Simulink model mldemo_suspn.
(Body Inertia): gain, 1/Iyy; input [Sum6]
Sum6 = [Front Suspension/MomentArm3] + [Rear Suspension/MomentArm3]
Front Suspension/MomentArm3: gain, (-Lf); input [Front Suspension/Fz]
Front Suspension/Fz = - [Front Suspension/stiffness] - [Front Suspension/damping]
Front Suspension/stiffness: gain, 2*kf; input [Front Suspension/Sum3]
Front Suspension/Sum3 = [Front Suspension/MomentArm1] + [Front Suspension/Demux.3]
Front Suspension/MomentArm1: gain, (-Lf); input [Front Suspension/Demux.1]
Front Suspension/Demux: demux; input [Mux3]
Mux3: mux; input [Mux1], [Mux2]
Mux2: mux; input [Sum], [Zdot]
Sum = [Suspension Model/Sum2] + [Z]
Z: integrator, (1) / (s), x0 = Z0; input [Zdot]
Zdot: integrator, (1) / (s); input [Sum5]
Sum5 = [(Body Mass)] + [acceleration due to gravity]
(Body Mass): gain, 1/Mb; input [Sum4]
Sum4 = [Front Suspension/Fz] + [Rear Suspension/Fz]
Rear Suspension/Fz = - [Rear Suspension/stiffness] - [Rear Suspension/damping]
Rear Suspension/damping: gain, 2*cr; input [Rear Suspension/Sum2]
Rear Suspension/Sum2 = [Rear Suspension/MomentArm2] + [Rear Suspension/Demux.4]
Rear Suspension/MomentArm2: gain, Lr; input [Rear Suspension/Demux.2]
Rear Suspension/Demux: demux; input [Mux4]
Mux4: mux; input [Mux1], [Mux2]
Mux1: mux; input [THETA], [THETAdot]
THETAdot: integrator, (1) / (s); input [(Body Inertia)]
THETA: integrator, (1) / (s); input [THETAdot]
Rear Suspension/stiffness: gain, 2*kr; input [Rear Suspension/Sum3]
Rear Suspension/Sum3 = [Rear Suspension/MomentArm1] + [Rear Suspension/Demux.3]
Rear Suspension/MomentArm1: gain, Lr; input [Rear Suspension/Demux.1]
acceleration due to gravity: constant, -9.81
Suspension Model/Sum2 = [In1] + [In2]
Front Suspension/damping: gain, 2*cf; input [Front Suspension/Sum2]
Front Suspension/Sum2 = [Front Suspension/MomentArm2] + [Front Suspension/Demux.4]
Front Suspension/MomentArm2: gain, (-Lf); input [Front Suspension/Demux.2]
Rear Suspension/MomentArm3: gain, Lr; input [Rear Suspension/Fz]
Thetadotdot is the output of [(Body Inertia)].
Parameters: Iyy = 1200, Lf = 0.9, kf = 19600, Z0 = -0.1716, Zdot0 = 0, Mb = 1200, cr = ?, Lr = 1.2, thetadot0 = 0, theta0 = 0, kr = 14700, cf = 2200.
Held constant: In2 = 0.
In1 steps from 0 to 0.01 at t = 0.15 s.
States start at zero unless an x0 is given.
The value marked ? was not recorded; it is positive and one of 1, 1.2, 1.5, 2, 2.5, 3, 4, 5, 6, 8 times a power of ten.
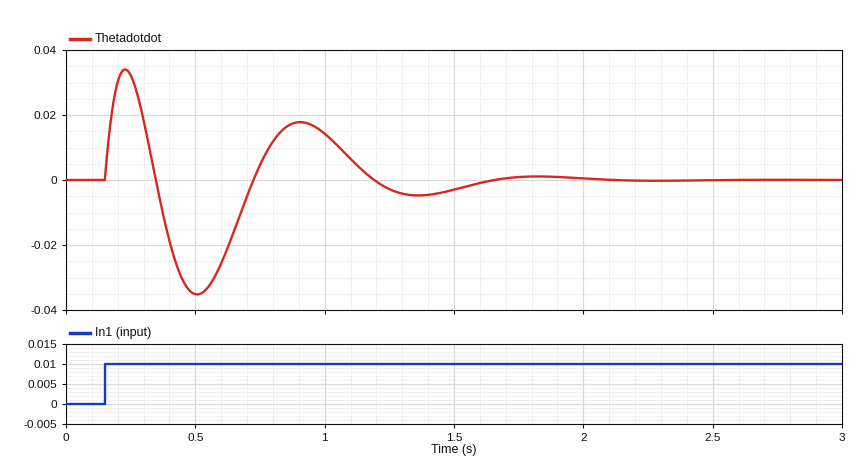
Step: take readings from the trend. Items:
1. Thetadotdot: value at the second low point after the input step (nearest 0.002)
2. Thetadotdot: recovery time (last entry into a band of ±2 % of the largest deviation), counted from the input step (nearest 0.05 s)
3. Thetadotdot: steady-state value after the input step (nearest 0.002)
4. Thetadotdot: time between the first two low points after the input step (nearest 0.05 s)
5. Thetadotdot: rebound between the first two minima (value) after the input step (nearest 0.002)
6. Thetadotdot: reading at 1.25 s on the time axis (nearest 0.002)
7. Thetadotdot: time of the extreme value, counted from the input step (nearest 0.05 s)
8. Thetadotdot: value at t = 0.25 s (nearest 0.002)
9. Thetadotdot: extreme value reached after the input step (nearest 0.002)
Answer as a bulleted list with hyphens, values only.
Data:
- -0.004
- 1.80 s
- 0.000
- 0.85 s
- 0.018
- -0.002
- 0.35 s
- 0.032
- -0.036
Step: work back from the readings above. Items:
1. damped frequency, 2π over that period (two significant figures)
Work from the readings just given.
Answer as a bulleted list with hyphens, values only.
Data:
- 7.4 rad/s
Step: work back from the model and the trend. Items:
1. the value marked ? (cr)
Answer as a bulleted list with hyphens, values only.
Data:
- 2500
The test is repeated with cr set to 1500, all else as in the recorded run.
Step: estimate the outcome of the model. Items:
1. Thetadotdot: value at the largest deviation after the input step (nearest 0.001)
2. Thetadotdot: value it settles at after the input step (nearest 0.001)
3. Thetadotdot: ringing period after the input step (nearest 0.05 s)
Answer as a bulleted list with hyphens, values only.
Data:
- 0.009
- 0.000
- 0.80 s
